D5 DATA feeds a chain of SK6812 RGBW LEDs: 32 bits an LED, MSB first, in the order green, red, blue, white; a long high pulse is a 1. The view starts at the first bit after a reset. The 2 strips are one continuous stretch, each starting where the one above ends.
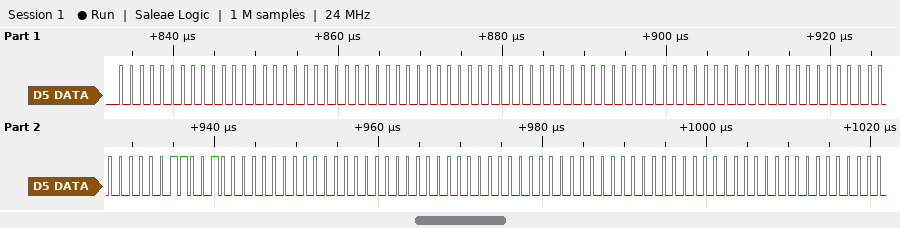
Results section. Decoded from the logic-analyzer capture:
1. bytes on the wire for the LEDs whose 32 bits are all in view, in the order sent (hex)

00 00 00 00 00 00 00 00 00 00 64 00 00 00 00 00
